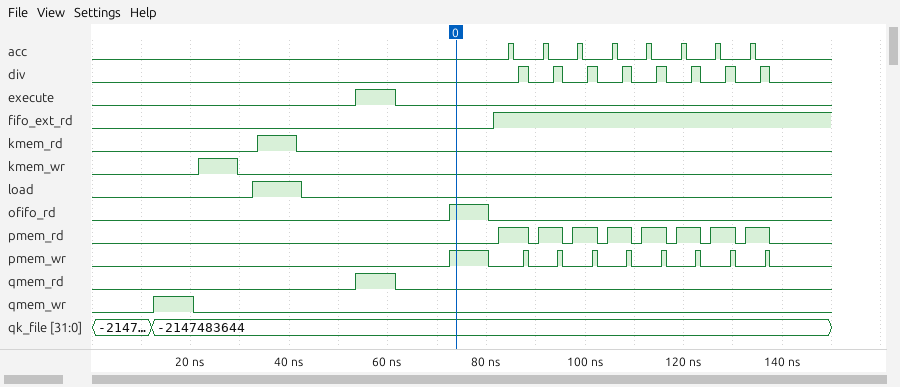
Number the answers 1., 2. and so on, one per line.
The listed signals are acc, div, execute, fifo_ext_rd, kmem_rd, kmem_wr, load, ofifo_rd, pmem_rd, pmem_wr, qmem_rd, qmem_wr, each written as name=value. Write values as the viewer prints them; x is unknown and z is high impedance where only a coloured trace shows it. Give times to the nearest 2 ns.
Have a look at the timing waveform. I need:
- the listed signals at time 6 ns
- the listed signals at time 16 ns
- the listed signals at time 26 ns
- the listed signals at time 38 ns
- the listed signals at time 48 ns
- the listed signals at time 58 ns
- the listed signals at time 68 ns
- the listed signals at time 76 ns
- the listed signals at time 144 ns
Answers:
1. acc=0, div=0, execute=0, fifo_ext_rd=0, kmem_rd=0, kmem_wr=0, load=0, ofifo_rd=0, pmem_rd=0, pmem_wr=0, qmem_rd=0, qmem_wr=0
2. acc=0, div=0, execute=0, fifo_ext_rd=0, kmem_rd=0, kmem_wr=0, load=0, ofifo_rd=0, pmem_rd=0, pmem_wr=0, qmem_rd=0, qmem_wr=1
3. acc=0, div=0, execute=0, fifo_ext_rd=0, kmem_rd=0, kmem_wr=1, load=0, ofifo_rd=0, pmem_rd=0, pmem_wr=0, qmem_rd=0, qmem_wr=0
4. acc=0, div=0, execute=0, fifo_ext_rd=0, kmem_rd=1, kmem_wr=0, load=1, ofifo_rd=0, pmem_rd=0, pmem_wr=0, qmem_rd=0, qmem_wr=0
5. acc=0, div=0, execute=0, fifo_ext_rd=0, kmem_rd=0, kmem_wr=0, load=0, ofifo_rd=0, pmem_rd=0, pmem_wr=0, qmem_rd=0, qmem_wr=0
6. acc=0, div=0, execute=1, fifo_ext_rd=0, kmem_rd=0, kmem_wr=0, load=0, ofifo_rd=0, pmem_rd=0, pmem_wr=0, qmem_rd=1, qmem_wr=0
7. acc=0, div=0, execute=0, fifo_ext_rd=0, kmem_rd=0, kmem_wr=0, load=0, ofifo_rd=0, pmem_rd=0, pmem_wr=0, qmem_rd=0, qmem_wr=0
8. acc=0, div=0, execute=0, fifo_ext_rd=0, kmem_rd=0, kmem_wr=0, load=0, ofifo_rd=1, pmem_rd=0, pmem_wr=1, qmem_rd=0, qmem_wr=0
9. acc=0, div=0, execute=0, fifo_ext_rd=1, kmem_rd=0, kmem_wr=0, load=0, ofifo_rd=0, pmem_rd=0, pmem_wr=0, qmem_rd=0, qmem_wr=0
